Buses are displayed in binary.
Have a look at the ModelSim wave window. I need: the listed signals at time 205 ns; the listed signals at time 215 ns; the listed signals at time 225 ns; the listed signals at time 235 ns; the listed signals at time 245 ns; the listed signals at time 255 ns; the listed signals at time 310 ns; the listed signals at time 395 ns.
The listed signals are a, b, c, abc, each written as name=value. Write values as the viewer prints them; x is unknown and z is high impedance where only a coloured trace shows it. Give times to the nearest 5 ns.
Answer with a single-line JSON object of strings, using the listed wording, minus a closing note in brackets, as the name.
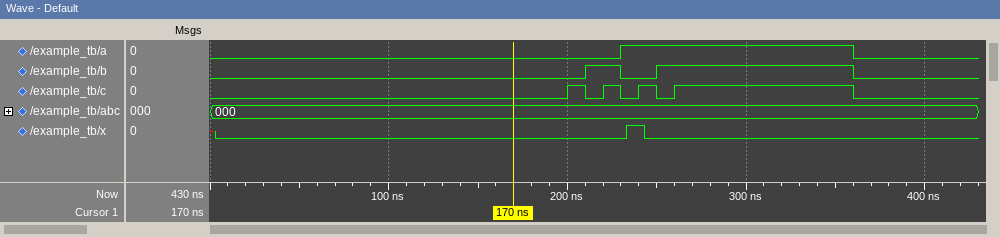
{"the listed signals at time 205 ns": "a=0, b=0, c=1, abc=000", "the listed signals at time 215 ns": "a=0, b=1, c=0, abc=000", "the listed signals at time 225 ns": "a=0, b=1, c=1, abc=000", "the listed signals at time 235 ns": "a=1, b=0, c=0, abc=000", "the listed signals at time 245 ns": "a=1, b=0, c=1, abc=000", "the listed signals at time 255 ns": "a=1, b=1, c=0, abc=000", "the listed signals at time 310 ns": "a=1, b=1, c=1, abc=000", "the listed signals at time 395 ns": "a=0, b=0, c=0, abc=000"}
